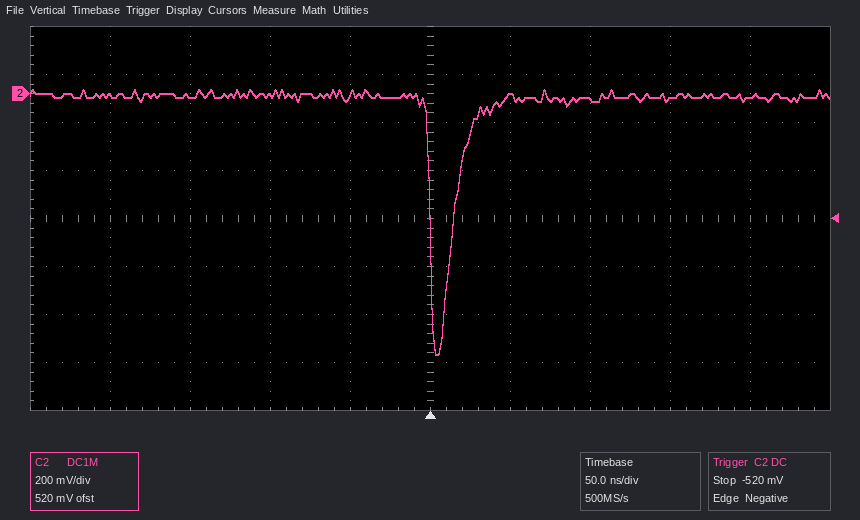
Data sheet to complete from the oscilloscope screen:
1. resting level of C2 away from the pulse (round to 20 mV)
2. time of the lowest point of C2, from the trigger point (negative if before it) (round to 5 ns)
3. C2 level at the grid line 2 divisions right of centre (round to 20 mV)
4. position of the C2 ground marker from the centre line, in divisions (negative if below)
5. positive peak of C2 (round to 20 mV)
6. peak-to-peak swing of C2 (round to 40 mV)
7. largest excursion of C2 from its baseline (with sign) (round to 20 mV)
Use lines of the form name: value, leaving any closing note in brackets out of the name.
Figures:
resting level of C2 away from the pulse: -20 mV
time of the lowest point of C2, from the trigger point (negative if before it): +5 ns
C2 level at the grid line 2 divisions right of centre: -20 mV
position of the C2 ground marker from the centre line, in divisions: +2.6 div
positive peak of C2: 20 mV
peak-to-peak swing of C2: 1.12 V
largest excursion of C2 from its baseline (with sign): -1.08 V
